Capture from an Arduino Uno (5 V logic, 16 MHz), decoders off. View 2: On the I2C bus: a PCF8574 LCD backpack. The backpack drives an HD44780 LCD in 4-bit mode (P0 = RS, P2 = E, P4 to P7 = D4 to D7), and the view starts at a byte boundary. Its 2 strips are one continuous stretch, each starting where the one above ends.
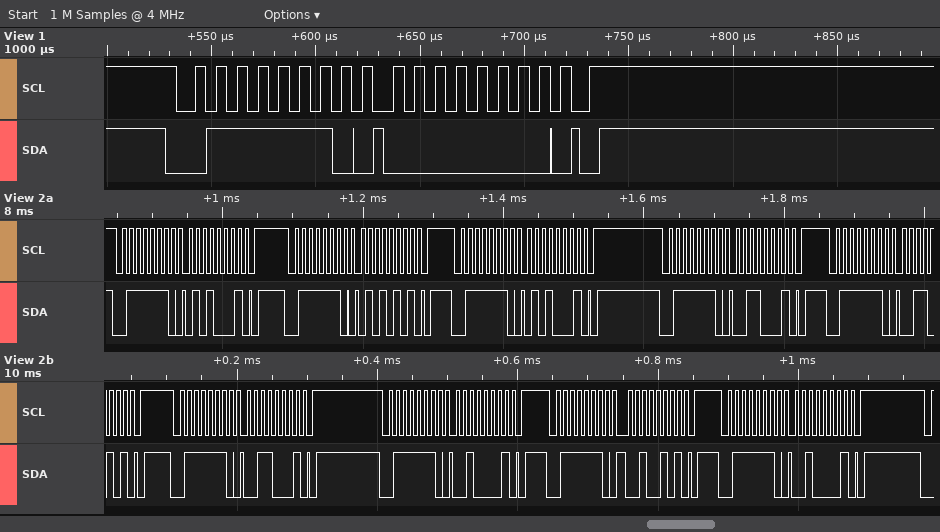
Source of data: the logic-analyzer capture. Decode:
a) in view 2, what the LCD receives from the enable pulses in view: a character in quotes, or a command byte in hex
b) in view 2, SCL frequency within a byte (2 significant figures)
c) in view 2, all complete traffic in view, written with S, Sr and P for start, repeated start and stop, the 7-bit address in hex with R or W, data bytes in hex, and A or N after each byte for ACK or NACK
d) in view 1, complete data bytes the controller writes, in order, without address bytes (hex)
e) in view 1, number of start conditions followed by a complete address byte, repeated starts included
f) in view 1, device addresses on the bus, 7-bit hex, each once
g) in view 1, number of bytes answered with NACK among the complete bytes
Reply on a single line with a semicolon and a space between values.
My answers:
'S'; 100 kHz; S 3FW A 51 A P S 3FW A 55 A P S 3FW A 51 A P S 3FW A 31 A P S 3FW A 35 A P S 3FW A 31 A P S 3FW A 21 A P S 3FW A 25 A P S 3FW A 21 A P; 00; 1; 0x3F; 0
